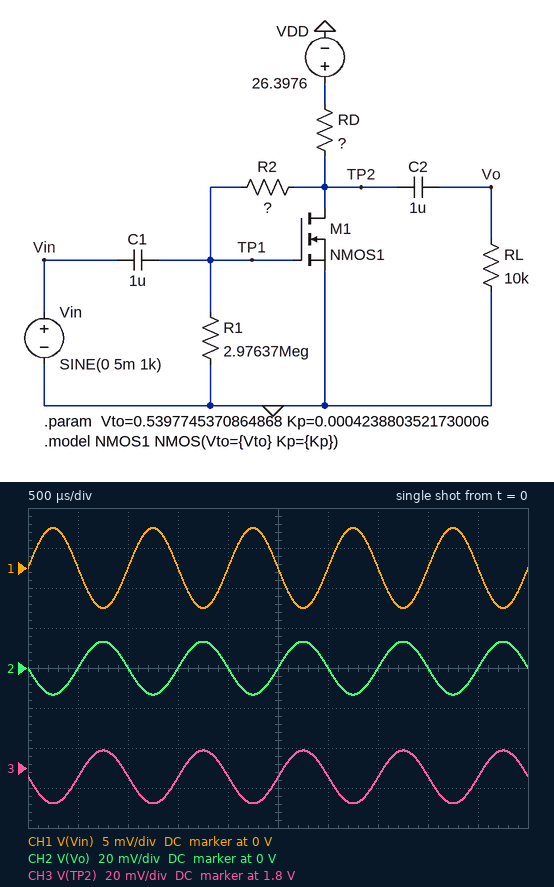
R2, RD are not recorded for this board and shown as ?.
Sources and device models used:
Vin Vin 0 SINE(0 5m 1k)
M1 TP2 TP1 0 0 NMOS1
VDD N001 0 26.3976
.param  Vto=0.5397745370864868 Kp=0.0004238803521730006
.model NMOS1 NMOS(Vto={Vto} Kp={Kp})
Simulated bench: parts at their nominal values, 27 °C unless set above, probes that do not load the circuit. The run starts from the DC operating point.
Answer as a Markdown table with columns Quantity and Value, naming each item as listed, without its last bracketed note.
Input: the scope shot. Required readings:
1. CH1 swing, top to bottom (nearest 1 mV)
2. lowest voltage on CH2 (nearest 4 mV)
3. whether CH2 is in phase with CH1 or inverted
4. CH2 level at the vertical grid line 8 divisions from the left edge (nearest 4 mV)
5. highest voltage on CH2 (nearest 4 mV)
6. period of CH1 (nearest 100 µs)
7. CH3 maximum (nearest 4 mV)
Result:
| Quantity | Value |
|---|---|
| CH1 swing, top to bottom | 10 mV |
| lowest voltage on CH2 | -12 mV |
| whether CH2 is in phase with CH1 or inverted | inverted |
| CH2 level at the vertical grid line 8 divisions from the left edge | 0 V |
| highest voltage on CH2 | 12 mV |
| period of CH1 | 1.0 ms |
| CH3 maximum | 1.808 V |
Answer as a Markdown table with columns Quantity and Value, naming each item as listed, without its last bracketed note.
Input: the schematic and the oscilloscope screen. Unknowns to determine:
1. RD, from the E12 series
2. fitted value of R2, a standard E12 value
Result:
| Quantity | Value |
|---|---|
| RD, from the E12 series | 270 kΩ |
| fitted value of R2, a standard E12 value | 1.5 MΩ |
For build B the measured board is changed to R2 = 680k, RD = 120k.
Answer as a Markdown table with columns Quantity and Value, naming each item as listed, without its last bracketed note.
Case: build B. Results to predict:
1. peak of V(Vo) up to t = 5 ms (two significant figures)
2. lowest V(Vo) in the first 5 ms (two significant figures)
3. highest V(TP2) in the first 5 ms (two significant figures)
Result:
| Quantity | Value |
|---|---|
| peak of V(Vo) up to t = 5 ms | 19 mV |
| lowest V(Vo) in the first 5 ms | -19 mV |
| highest V(TP2) in the first 5 ms | 1.9 V |
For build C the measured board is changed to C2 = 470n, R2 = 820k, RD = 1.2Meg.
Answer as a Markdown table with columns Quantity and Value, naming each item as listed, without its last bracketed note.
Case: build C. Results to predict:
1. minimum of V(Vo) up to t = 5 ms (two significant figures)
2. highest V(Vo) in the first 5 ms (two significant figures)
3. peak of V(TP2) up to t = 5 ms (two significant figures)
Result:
| Quantity | Value |
|---|---|
| minimum of V(Vo) up to t = 5 ms | -6.5 mV |
| highest V(Vo) in the first 5 ms | 6.4 mV |
| peak of V(TP2) up to t = 5 ms | 1.1 V |
